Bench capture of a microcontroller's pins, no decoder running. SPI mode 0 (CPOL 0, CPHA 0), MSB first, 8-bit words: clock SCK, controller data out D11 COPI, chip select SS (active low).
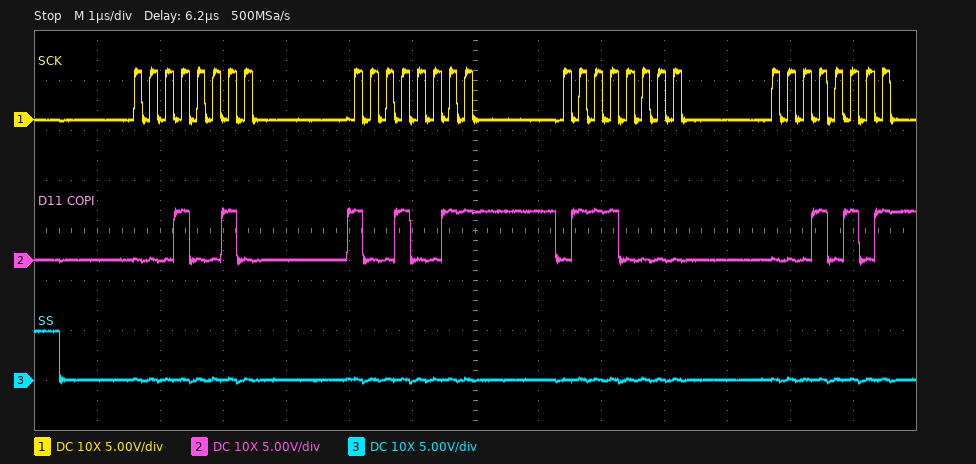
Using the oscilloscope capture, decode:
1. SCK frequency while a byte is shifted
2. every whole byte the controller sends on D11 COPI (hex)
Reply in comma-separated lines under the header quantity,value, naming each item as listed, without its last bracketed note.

quantity,value
SCK frequency while a byte is shifted,4 MHz
every whole byte the controller sends on D11 COPI,12 93 70 15
